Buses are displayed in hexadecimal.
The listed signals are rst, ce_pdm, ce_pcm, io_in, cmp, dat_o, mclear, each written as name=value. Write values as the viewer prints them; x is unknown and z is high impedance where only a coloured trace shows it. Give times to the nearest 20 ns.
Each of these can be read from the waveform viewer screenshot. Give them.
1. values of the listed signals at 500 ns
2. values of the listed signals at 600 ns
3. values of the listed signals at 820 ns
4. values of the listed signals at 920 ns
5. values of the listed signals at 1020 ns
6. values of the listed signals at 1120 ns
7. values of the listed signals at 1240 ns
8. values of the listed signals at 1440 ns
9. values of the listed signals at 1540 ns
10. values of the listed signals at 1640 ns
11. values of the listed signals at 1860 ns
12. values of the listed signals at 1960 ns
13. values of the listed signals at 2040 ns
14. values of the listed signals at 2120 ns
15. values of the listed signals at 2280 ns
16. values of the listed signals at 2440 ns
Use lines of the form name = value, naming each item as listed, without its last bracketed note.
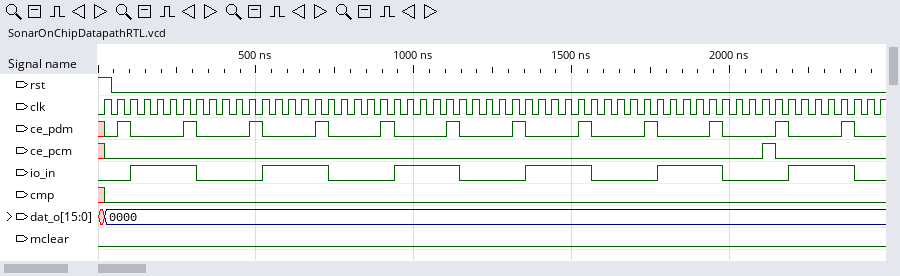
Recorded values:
values of the listed signals at 500 ns = rst=0, ce_pdm=1, ce_pcm=0, io_in=0, cmp=0, dat_o=0000, mclear=0
values of the listed signals at 600 ns = rst=0, ce_pdm=0, ce_pcm=0, io_in=1, cmp=0, dat_o=0000, mclear=0
values of the listed signals at 820 ns = rst=0, ce_pdm=0, ce_pcm=0, io_in=0, cmp=0, dat_o=0000, mclear=0
values of the listed signals at 920 ns = rst=0, ce_pdm=1, ce_pcm=0, io_in=0, cmp=0, dat_o=0000, mclear=0
values of the listed signals at 1020 ns = rst=0, ce_pdm=0, ce_pcm=0, io_in=1, cmp=0, dat_o=0000, mclear=0
values of the listed signals at 1120 ns = rst=0, ce_pdm=1, ce_pcm=0, io_in=1, cmp=0, dat_o=0000, mclear=0
values of the listed signals at 1240 ns = rst=0, ce_pdm=0, ce_pcm=0, io_in=0, cmp=0, dat_o=0000, mclear=0
values of the listed signals at 1440 ns = rst=0, ce_pdm=0, ce_pcm=0, io_in=1, cmp=0, dat_o=0000, mclear=0
values of the listed signals at 1540 ns = rst=0, ce_pdm=1, ce_pcm=0, io_in=1, cmp=0, dat_o=0000, mclear=0
values of the listed signals at 1640 ns = rst=0, ce_pdm=0, ce_pcm=0, io_in=0, cmp=0, dat_o=0000, mclear=0
values of the listed signals at 1860 ns = rst=0, ce_pdm=0, ce_pcm=0, io_in=1, cmp=0, dat_o=0000, mclear=0
values of the listed signals at 1960 ns = rst=0, ce_pdm=1, ce_pcm=0, io_in=1, cmp=0, dat_o=0000, mclear=0
values of the listed signals at 2040 ns = rst=0, ce_pdm=0, ce_pcm=0, io_in=0, cmp=0, dat_o=0000, mclear=0
values of the listed signals at 2120 ns = rst=0, ce_pdm=0, ce_pcm=1, io_in=0, cmp=0, dat_o=0000, mclear=0
values of the listed signals at 2280 ns = rst=0, ce_pdm=0, ce_pcm=0, io_in=1, cmp=0, dat_o=0000, mclear=0
values of the listed signals at 2440 ns = rst=0, ce_pdm=0, ce_pcm=0, io_in=0, cmp=0, dat_o=0000, mclear=0
